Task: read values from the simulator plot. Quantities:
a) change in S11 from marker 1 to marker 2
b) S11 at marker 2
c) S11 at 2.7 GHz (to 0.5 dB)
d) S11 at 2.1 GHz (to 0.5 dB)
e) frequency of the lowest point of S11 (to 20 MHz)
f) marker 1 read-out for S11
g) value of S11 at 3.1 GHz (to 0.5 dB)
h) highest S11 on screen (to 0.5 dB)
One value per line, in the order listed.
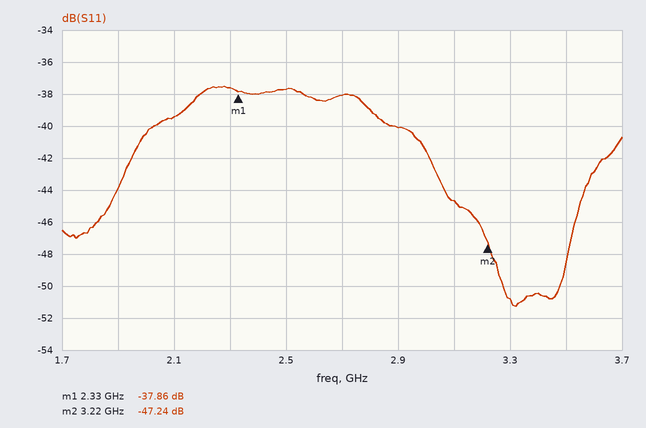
-9.38 dB
-47.24 dB
-38.0 dB
-39.5 dB
3.32 GHz
-37.86 dB
-44.5 dB
-37.5 dB
